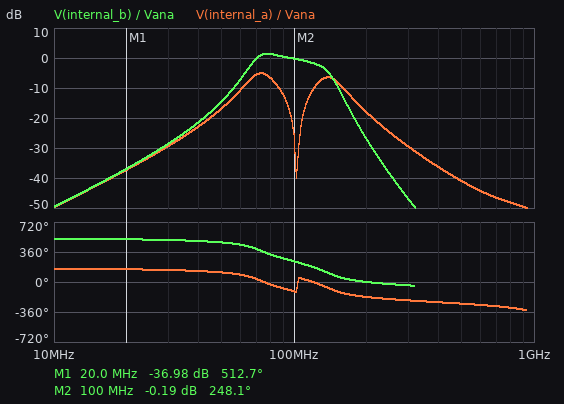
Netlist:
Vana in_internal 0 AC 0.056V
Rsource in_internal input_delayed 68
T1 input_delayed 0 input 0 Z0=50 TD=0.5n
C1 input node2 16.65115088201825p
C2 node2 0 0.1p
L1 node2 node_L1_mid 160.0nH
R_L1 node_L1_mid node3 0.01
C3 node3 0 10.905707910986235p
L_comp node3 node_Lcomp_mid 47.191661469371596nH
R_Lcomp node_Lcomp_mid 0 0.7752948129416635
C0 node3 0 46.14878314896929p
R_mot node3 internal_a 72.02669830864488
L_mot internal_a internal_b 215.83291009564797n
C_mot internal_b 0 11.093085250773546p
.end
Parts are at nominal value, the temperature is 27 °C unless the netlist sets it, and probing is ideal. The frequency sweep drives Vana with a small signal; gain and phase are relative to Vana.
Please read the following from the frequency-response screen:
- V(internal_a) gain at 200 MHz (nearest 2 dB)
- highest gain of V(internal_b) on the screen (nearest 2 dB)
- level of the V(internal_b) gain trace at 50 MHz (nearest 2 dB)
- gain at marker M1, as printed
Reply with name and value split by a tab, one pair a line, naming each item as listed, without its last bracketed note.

V(internal_a) gain at 200 MHz	-18 dB
highest gain of V(internal_b) on the screen	2 dB
level of the V(internal_b) gain trace at 50 MHz	-14 dB
gain at marker M1, as printed	-36.98 dB
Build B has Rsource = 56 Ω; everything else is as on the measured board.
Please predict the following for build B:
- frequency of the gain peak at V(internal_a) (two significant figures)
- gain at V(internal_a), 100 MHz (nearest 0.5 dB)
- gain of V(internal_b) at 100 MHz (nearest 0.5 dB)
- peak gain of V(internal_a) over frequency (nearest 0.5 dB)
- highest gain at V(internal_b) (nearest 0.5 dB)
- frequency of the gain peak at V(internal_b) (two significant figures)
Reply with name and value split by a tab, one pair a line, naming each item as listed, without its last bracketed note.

frequency of the gain peak at V(internal_a)	72 MHz
gain at V(internal_a), 100 MHz	-24.5 dB
gain of V(internal_b) at 100 MHz	0.5 dB
peak gain of V(internal_a) over frequency	-4.0 dB
highest gain at V(internal_b)	2.5 dB
frequency of the gain peak at V(internal_b)	76 MHz
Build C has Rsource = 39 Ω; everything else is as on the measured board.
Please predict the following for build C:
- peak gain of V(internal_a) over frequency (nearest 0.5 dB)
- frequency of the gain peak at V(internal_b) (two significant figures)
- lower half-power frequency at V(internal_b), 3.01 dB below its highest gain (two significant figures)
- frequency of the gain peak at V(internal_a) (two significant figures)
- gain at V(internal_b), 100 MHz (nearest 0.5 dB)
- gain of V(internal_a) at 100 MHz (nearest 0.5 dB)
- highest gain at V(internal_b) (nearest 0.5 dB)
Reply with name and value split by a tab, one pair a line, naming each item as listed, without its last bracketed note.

peak gain of V(internal_a) over frequency	-2.0 dB
frequency of the gain peak at V(internal_b)	73 MHz
lower half-power frequency at V(internal_b), 3.01 dB below its highest gain	66 MHz
frequency of the gain peak at V(internal_a)	71 MHz
gain at V(internal_b), 100 MHz	2.0 dB
gain of V(internal_a) at 100 MHz	-23.0 dB
highest gain at V(internal_b)	4.0 dB
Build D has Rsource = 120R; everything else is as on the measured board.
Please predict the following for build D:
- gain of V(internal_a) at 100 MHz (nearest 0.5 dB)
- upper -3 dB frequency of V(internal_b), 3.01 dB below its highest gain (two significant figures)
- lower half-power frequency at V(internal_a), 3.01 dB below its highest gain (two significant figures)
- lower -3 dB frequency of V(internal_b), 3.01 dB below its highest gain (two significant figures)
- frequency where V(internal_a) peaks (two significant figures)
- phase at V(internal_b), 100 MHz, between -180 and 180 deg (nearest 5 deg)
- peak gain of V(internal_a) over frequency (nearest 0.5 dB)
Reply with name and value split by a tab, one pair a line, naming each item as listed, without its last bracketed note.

gain of V(internal_a) at 100 MHz	-28.5 dB
upper -3 dB frequency of V(internal_b), 3.01 dB below its highest gain	110 MHz
lower half-power frequency at V(internal_a), 3.01 dB below its highest gain	66 MHz
lower -3 dB frequency of V(internal_b), 3.01 dB below its highest gain	70 MHz
frequency where V(internal_a) peaks	75 MHz
phase at V(internal_b), 100 MHz, between -180 and 180 deg	-115 deg
peak gain of V(internal_a) over frequency	-8.5 dB
